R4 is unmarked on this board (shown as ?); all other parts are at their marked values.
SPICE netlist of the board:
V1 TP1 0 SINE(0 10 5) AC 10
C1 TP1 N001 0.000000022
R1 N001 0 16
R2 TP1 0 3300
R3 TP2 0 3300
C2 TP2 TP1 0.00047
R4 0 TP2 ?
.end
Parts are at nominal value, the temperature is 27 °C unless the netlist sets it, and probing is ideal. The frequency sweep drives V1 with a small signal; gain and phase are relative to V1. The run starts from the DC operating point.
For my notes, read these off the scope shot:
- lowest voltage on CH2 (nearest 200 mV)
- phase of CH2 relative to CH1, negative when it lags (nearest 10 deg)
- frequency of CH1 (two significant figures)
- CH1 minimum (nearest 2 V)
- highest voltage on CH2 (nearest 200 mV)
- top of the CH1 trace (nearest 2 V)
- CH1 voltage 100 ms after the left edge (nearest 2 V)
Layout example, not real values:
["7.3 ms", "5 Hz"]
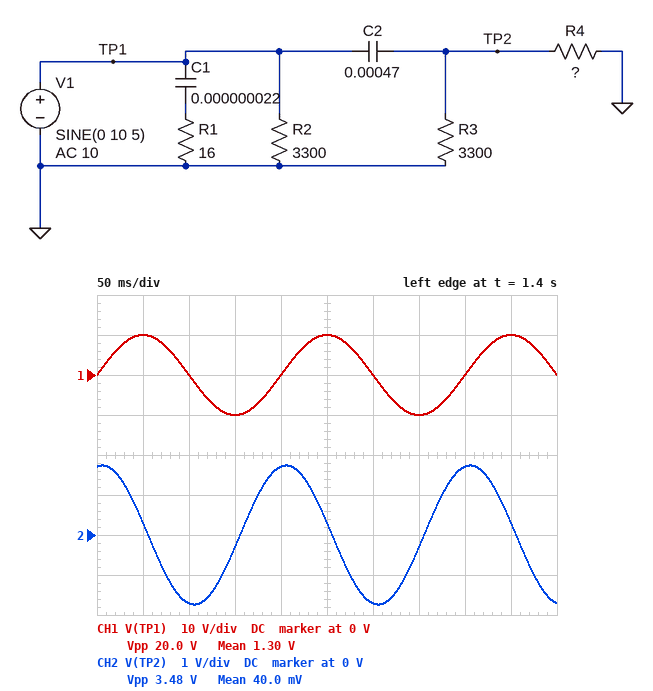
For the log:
["-1.8 V", "80 deg", "5.0 Hz", "-10 V", "1.8 V", "10 V", "0 V"]
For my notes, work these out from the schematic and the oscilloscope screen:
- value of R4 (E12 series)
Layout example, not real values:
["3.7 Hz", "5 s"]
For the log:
["12 Ω"]
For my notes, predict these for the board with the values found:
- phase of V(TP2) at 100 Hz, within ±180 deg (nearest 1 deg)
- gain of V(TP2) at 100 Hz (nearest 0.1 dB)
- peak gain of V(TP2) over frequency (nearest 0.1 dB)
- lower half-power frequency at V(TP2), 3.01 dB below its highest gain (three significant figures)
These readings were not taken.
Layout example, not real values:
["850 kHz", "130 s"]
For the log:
["16 deg", "-0.3 dB", "0 dB", "28.3 Hz"]
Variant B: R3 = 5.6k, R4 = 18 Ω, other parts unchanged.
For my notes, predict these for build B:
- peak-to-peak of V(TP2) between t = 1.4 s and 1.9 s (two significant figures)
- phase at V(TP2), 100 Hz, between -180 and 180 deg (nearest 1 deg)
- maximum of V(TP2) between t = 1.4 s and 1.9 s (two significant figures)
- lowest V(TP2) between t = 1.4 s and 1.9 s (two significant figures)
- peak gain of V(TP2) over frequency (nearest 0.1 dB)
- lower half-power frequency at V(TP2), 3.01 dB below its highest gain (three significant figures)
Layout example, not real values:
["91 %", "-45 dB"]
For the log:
["5.1 V", "11 deg", "2.6 V", "-2.6 V", "0 dB", "18.9 Hz"]
